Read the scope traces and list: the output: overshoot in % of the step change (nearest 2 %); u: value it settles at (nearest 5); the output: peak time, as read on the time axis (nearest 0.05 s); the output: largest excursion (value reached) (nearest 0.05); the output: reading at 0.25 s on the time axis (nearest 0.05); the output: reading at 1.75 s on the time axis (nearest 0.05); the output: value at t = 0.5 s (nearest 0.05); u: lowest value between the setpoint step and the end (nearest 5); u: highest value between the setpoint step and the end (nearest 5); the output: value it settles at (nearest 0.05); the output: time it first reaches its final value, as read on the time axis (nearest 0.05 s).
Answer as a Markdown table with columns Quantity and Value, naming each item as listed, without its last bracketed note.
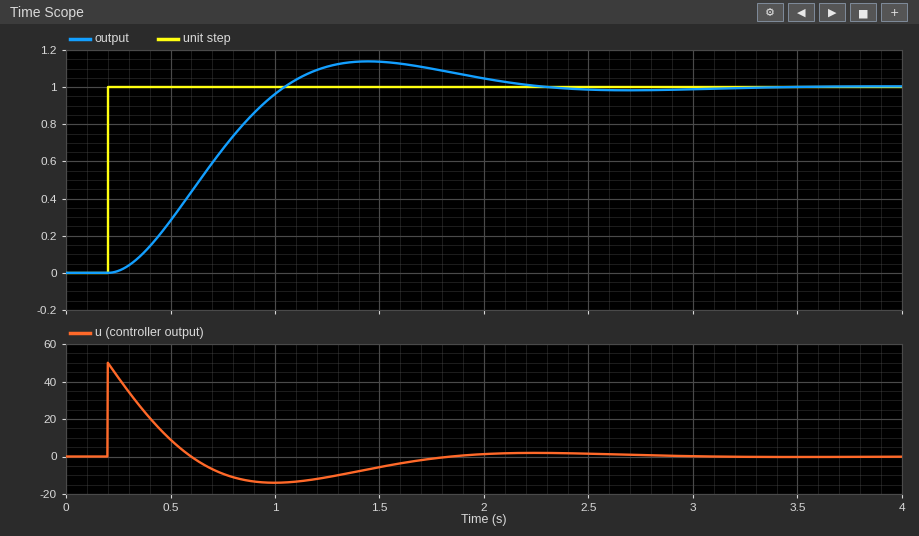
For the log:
| Quantity | Value |
|---|---|
| the output: overshoot in % of the step change | 14 % |
| u: value it settles at | 0 |
| the output: peak time, as read on the time axis | 1.45 s |
| the output: largest excursion (value reached) | 1.15 |
| the output: reading at 0.25 s on the time axis | 0.00 |
| the output: reading at 1.75 s on the time axis | 1.10 |
| the output: value at t = 0.5 s | 0.30 |
| u: lowest value between the setpoint step and the end | -15 |
| u: highest value between the setpoint step and the end | 50 |
| the output: value it settles at | 1.00 |
| the output: time it first reaches its final value, as read on the time axis | 1.05 s |
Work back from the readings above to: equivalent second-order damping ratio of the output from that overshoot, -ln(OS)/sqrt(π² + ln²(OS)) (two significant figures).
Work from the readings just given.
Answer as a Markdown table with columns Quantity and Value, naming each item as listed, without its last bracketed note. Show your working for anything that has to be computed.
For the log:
| Quantity | Value |
|---|---|
| equivalent second-order damping ratio of the output from that overshoot, -ln(OS)/sqrt(π² + ln²(OS)) | ln(0.14) = -1.966; 1.966 / sqrt(9.870 + 3.866) = 0.53 |
